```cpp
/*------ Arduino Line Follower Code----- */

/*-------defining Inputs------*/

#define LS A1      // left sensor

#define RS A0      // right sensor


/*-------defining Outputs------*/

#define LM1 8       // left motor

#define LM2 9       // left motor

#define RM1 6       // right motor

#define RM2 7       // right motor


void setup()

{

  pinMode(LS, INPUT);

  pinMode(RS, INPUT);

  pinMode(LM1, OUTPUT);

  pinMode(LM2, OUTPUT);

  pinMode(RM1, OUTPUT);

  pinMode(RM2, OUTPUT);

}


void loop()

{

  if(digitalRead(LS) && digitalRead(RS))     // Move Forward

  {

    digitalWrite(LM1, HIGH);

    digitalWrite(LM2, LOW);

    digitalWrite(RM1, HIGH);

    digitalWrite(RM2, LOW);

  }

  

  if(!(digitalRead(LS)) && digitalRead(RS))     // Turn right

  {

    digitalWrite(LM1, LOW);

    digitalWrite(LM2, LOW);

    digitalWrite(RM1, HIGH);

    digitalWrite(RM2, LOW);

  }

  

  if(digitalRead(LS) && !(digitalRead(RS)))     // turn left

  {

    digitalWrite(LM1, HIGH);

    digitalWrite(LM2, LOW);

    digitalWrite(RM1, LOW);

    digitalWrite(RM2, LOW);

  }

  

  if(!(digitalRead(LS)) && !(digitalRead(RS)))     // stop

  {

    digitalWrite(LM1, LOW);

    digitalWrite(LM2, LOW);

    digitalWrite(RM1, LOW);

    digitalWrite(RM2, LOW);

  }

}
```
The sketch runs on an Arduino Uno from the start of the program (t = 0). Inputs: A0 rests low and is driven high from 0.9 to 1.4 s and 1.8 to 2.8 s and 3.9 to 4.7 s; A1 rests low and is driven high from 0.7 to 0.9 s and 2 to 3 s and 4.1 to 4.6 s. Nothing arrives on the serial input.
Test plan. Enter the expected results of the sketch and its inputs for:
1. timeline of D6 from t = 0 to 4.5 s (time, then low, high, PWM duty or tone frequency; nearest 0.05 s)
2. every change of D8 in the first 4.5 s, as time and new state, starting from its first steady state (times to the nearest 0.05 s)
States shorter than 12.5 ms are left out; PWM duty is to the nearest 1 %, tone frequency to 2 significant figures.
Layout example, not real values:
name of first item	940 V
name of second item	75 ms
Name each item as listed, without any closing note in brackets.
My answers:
timeline of D6 from t = 0 to 4.5 s	0 s low; 0.9 s high; 1.4 s low; 1.8 s high; 2.8 s low; 3.9 s high
every change of D8 in the first 4.5 s, as time and new state, starting from its first steady state	0 s low; 0.7 s high; 0.9 s low; 2 s high; 3 s low; 4.1 s high
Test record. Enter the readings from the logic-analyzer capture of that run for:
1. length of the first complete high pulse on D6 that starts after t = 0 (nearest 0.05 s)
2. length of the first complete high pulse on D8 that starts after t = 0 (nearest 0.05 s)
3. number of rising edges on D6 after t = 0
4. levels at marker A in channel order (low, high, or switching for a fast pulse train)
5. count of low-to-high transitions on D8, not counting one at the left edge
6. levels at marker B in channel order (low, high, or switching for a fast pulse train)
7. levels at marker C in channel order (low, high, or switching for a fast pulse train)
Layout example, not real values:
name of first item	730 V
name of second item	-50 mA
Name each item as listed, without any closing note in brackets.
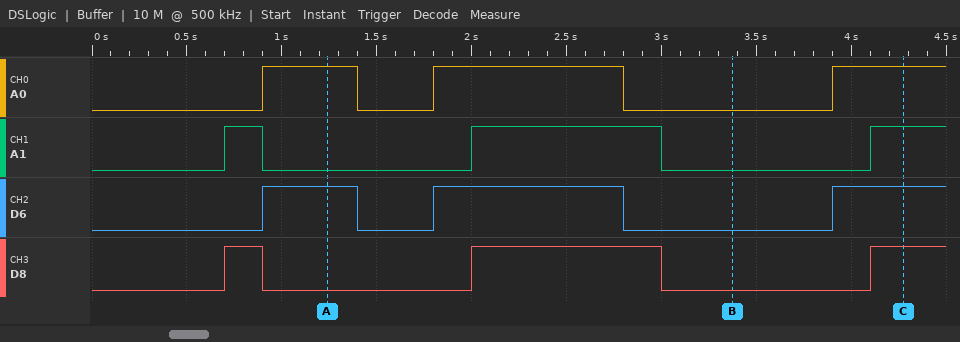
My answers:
length of the first complete high pulse on D6 that starts after t = 0	0.50 s
length of the first complete high pulse on D8 that starts after t = 0	0.20 s
number of rising edges on D6 after t = 0	3
levels at marker A in channel order	A0 high, A1 low, D6 high, D8 low
count of low-to-high transitions on D8, not counting one at the left edge	3
levels at marker B in channel order	A0 low, A1 low, D6 low, D8 low
levels at marker C in channel order	A0 high, A1 high, D6 high, D8 high
